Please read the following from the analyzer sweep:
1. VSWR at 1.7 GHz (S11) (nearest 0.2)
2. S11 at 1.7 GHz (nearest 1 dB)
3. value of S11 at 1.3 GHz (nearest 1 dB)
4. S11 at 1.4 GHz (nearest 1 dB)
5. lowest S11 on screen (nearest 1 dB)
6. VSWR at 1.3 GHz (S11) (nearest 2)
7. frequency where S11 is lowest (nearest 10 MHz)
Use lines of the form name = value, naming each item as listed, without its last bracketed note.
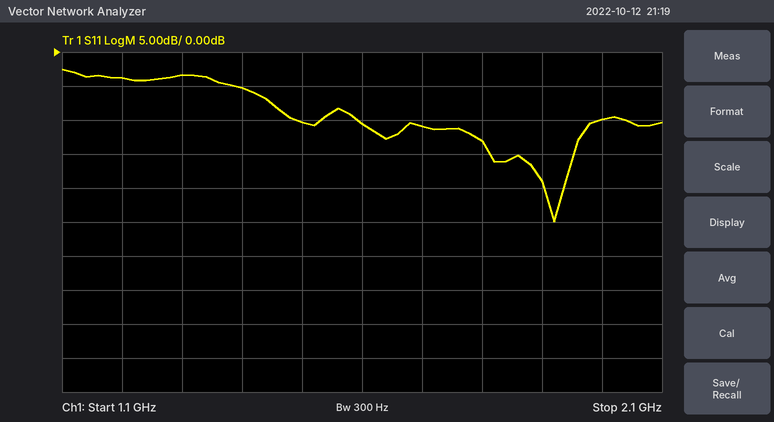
VSWR at 1.7 GHz (S11) = 1.8
S11 at 1.7 GHz = -11 dB
value of S11 at 1.3 GHz = -3 dB
S11 at 1.4 GHz = -5 dB
lowest S11 on screen = -25 dB
VSWR at 1.3 GHz (S11) = 6
frequency where S11 is lowest = 1.92 GHz
